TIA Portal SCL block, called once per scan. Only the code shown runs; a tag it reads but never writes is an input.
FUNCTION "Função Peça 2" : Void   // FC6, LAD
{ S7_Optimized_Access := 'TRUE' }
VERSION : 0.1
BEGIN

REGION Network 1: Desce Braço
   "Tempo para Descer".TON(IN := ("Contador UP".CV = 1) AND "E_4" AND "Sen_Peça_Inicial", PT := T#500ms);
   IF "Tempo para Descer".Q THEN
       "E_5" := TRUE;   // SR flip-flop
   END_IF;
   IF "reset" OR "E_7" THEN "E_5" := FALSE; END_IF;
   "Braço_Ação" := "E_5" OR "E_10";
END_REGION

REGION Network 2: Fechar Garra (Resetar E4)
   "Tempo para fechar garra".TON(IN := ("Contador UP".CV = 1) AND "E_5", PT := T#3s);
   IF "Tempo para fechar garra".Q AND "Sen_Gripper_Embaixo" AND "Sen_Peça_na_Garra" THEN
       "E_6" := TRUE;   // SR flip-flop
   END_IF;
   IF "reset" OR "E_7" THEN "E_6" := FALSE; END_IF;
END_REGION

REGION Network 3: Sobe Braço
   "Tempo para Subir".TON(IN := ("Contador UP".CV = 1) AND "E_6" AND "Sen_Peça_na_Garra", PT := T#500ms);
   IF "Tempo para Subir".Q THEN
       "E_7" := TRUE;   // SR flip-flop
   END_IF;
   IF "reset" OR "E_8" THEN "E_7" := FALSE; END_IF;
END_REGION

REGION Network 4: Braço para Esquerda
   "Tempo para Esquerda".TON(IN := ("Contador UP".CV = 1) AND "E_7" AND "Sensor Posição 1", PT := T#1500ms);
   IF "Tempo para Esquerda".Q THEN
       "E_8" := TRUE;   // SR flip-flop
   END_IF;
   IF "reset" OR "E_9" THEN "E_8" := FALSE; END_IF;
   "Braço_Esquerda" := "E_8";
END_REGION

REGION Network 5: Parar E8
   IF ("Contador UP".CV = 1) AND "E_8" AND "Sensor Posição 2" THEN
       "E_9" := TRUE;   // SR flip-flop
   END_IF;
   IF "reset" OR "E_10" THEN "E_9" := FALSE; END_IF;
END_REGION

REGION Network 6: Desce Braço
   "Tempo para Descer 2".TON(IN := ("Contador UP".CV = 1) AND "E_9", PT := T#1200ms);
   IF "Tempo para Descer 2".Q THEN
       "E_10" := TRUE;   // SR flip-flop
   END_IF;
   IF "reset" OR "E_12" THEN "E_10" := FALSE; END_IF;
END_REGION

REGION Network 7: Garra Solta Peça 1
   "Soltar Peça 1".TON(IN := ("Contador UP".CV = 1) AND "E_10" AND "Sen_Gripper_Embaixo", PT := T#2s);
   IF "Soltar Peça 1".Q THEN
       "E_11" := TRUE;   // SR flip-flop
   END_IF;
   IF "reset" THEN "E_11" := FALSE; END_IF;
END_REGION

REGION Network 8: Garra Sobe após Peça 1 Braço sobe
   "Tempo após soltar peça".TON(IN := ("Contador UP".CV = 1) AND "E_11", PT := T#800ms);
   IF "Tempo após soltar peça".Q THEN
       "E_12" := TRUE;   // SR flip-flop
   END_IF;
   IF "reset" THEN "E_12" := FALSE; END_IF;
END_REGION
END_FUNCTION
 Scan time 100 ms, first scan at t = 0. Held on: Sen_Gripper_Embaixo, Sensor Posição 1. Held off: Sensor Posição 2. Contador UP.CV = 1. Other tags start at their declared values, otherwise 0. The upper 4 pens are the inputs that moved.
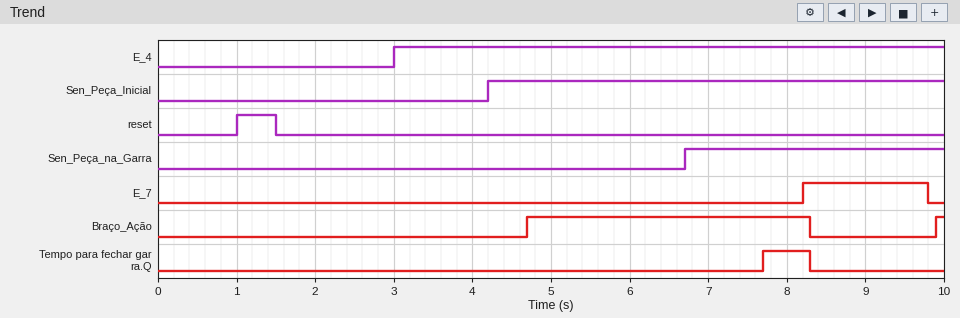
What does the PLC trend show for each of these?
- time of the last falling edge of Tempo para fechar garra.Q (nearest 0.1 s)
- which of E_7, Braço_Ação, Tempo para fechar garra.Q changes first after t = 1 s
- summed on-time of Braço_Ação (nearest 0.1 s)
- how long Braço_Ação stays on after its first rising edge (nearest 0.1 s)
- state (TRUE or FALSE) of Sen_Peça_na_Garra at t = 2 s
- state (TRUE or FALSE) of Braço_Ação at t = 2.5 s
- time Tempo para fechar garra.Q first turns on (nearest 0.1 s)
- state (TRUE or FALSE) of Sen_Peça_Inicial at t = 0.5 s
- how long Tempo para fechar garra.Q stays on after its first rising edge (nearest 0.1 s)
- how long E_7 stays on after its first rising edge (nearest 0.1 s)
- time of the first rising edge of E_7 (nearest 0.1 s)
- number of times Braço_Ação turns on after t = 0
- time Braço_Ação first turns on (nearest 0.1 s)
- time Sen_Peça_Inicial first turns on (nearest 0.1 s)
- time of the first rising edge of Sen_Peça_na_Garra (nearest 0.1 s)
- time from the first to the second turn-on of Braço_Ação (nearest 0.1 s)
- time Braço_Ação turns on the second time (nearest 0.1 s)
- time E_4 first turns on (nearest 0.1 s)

8.3 s
Braço_Ação
3.7 s
3.6 s
FALSE
FALSE
7.7 s
FALSE
0.6 s
1.6 s
8.2 s
2
4.7 s
4.2 s
6.7 s
5.2 s
9.9 s
3.0 s
